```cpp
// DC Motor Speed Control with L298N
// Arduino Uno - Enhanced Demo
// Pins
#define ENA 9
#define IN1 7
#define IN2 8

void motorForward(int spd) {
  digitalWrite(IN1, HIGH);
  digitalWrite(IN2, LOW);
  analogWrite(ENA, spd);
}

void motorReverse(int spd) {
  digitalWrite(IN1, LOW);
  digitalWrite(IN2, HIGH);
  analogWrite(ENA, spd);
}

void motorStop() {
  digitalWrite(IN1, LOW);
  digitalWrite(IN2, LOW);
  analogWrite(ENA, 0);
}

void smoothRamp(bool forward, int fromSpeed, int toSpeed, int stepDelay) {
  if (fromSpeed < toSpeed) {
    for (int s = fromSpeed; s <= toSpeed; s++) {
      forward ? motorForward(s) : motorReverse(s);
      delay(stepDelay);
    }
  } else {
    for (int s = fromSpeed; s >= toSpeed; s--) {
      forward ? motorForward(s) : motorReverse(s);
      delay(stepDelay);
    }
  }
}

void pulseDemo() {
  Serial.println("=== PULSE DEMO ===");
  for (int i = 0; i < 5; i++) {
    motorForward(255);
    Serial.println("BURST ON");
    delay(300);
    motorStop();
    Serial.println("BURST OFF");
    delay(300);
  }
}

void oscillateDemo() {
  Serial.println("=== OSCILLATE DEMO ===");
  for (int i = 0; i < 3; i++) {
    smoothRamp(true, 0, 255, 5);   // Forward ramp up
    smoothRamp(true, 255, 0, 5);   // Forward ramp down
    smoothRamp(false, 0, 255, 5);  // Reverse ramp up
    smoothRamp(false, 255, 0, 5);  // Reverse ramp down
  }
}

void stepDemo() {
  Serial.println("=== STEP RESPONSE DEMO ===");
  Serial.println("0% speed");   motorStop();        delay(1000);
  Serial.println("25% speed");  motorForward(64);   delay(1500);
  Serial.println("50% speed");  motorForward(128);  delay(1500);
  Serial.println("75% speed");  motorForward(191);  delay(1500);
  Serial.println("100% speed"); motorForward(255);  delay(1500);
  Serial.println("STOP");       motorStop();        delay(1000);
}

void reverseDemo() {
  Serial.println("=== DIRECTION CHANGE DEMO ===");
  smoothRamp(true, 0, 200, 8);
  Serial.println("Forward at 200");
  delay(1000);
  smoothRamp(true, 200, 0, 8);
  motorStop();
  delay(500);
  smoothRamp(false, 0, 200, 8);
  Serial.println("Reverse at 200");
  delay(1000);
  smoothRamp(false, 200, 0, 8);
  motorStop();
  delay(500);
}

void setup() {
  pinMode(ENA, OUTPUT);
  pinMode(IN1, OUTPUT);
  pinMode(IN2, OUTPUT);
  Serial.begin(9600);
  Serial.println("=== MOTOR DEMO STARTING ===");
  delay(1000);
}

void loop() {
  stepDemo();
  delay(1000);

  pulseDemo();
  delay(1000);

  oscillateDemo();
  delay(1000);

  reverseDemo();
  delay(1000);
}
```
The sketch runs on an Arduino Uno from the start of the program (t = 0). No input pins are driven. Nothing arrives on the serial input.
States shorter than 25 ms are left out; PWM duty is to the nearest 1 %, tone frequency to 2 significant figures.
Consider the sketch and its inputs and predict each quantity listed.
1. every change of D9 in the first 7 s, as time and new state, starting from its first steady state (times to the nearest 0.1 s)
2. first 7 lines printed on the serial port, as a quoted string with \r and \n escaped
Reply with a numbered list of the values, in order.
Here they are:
1. 0 s low; 2 s PWM 25 %; 3.5 s PWM 50 %; 5 s PWM 75 %; 6.5 s high
2. "=== MOTOR DEMO STARTING ===\r\n=== STEP RESPONSE DEMO ===\r\n0% speed\r\n25% speed\r\n50% speed\r\n75% speed\r\n100% speed\r\n"
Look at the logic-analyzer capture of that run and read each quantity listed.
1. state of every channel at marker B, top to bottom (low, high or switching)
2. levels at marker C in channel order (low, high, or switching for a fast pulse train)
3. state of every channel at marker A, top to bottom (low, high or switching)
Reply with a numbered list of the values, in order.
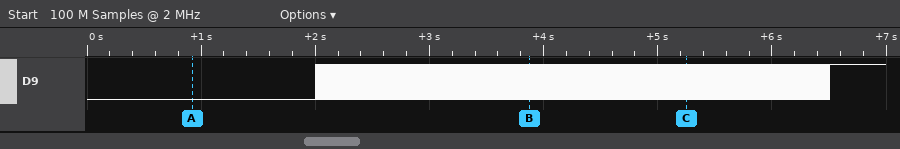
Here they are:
1. D9 switching
2. D9 switching
3. D9 low
